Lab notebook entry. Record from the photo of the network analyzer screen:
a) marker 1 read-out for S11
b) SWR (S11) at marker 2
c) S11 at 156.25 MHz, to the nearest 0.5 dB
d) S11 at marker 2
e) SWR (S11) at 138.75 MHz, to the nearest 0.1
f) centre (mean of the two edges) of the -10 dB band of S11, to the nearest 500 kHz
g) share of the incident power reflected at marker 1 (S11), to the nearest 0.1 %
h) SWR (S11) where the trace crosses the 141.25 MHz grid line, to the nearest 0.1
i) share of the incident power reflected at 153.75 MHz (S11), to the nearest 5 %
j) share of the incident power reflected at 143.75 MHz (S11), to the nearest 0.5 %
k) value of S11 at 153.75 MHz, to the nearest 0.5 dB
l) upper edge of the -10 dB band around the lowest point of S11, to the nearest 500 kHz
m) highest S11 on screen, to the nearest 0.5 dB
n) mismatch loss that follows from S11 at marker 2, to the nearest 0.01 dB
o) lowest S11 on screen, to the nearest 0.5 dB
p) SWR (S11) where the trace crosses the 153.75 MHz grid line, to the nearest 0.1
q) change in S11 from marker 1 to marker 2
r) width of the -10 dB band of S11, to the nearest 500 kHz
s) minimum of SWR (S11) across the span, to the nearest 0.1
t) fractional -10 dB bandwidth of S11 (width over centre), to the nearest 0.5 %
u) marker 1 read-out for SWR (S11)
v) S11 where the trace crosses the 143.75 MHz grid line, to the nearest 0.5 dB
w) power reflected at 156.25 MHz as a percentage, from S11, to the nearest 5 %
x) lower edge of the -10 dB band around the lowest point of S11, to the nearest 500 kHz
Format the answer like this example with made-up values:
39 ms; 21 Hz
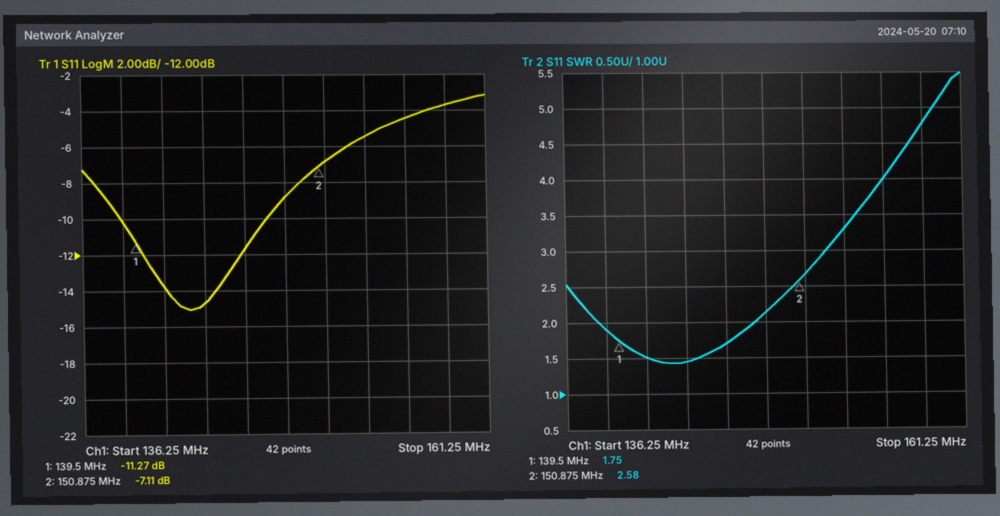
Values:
-11.27 dB; 2.58; -4.5 dB; -7.11 dB; 1.9; 143.0 MHz; 7.5 %; 1.5; 30 %; 3.5 %; -5.5 dB; 147.5 MHz; -3.0 dB; 0.94 dB; -15.0 dB; 3.3; 4.16 dB; 9.0 MHz; 1.4; 6.5 %; 1.75; -14.5 dB; 35 %; 138.5 MHz
